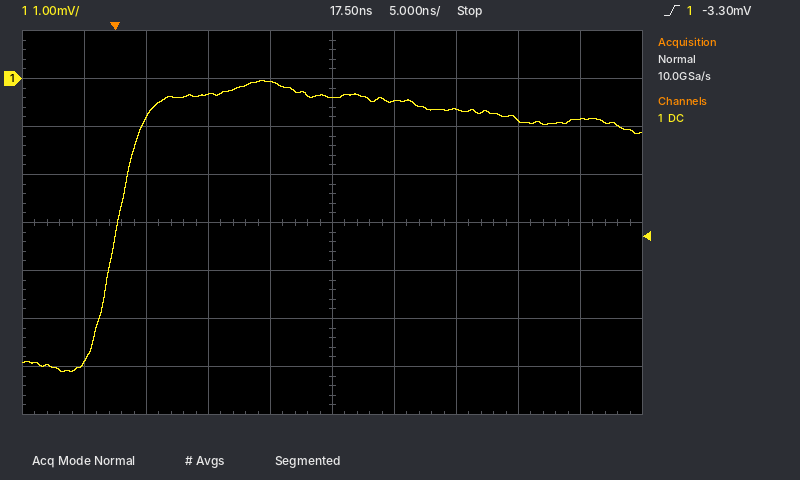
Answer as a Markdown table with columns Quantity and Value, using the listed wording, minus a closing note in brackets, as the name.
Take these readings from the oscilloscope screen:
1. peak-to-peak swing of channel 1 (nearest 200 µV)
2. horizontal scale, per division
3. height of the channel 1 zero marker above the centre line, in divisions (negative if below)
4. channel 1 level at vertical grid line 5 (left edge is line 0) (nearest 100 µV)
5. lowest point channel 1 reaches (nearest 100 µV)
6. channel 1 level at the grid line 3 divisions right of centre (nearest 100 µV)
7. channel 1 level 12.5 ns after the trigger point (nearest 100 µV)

| Quantity | Value |
|---|---|
| peak-to-peak swing of channel 1 | 6.0 mV |
| horizontal scale, per division | 5 ns |
| height of the channel 1 zero marker above the centre line, in divisions | +3.0 div |
| channel 1 level at vertical grid line 5 (left edge is line 0) | -400 µV |
| lowest point channel 1 reaches | -6.1 mV |
| channel 1 level at the grid line 3 divisions right of centre | -900 µV |
| channel 1 level 12.5 ns after the trigger point | -100 µV |
